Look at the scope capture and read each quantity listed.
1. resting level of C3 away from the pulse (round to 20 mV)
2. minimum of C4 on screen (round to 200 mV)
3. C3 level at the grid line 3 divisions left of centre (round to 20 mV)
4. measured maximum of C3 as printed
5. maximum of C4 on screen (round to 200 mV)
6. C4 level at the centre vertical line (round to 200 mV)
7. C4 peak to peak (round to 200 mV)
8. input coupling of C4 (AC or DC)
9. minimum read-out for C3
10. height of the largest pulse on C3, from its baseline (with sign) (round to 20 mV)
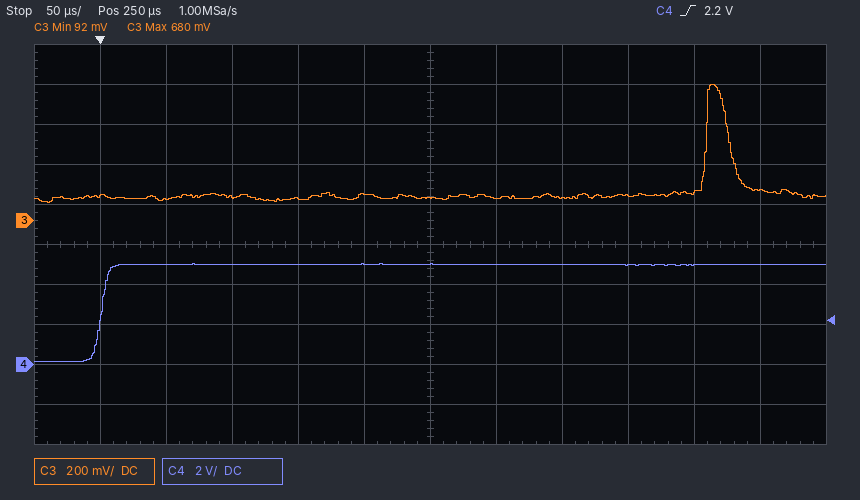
120 mV
200 mV
120 mV
680 mV
5.0 V
5.0 V
4.8 V
DC
92 mV
+560 mV
